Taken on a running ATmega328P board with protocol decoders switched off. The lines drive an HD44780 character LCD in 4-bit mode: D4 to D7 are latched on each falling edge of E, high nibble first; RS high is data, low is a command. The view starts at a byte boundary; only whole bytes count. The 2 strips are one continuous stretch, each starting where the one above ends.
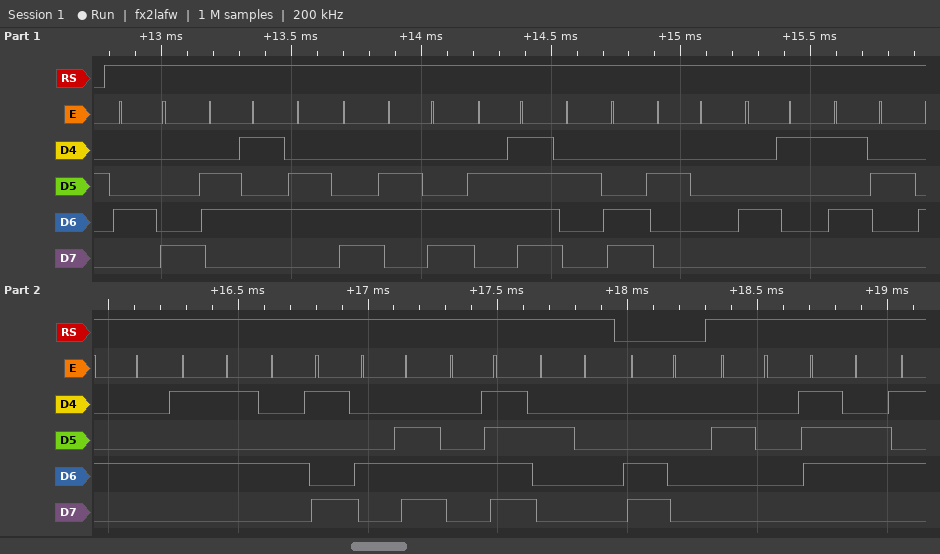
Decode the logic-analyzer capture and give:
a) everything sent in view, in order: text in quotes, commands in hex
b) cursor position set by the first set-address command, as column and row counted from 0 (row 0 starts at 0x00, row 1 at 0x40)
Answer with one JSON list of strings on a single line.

["\"Hello, ARDUINO \" 0xC0 \" v\"", "column 0, row 1"]
